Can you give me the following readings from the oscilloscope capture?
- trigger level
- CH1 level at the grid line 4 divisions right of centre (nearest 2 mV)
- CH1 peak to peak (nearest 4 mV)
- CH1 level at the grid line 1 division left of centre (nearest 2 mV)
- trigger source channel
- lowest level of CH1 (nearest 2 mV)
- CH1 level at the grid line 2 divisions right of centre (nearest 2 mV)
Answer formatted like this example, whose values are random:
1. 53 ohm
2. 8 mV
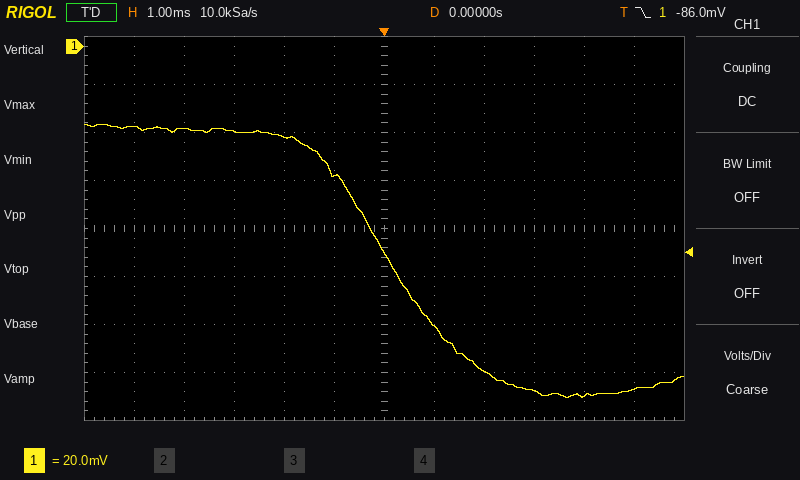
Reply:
1. -86.0 mV
2. -146 mV
3. 112 mV
4. -54 mV
5. CH1
6. -146 mV
7. -136 mV
